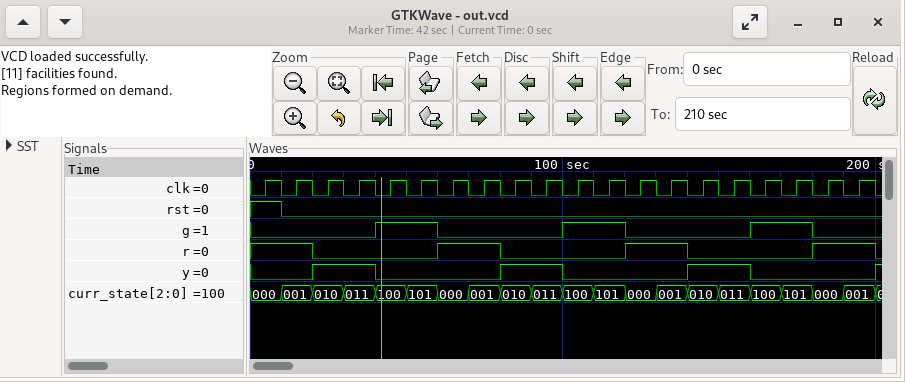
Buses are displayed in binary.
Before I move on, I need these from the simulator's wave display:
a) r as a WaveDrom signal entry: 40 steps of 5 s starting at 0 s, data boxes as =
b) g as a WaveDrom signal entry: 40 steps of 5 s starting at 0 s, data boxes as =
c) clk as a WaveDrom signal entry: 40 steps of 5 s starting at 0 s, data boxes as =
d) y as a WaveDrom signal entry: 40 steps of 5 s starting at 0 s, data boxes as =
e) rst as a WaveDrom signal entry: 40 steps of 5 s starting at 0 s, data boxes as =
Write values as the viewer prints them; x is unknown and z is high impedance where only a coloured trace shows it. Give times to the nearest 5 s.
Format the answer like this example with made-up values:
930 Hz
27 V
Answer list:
{name: 'r', wave: '1...0.......1...0.......1...0.......1...'}
{name: 'g', wave: '0.......1...0.......1...0.......1...0...'}
{name: 'clk', wave: '0101010101010101010101010101010101010101'}
{name: 'y', wave: '0...1...0.......1...0.......1...0.......'}
{name: 'rst', wave: '1.0.....................................'}
